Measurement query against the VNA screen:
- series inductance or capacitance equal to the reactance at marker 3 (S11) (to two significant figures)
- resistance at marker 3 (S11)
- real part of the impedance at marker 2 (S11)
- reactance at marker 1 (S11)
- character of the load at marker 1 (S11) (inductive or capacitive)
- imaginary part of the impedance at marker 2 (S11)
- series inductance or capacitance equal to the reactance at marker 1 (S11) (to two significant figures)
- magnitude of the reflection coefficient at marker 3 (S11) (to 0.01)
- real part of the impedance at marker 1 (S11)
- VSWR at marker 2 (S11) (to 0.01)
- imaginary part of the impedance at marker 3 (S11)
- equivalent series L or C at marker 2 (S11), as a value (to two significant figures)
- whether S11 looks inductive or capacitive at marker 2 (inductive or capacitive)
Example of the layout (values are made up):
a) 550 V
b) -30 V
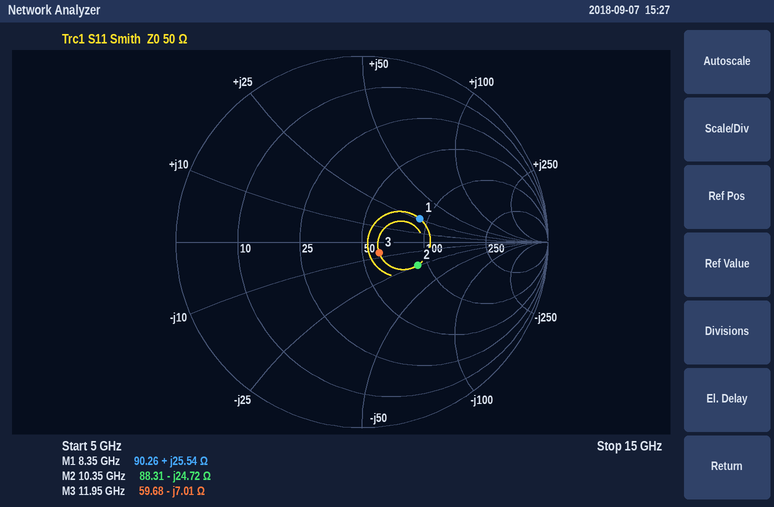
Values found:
a) 1.9 pF
b) 59.68 Ω
c) 88.31 Ω
d) +25.54 Ω
e) inductive
f) -24.72 Ω
g) 490 pH
h) 0.11
i) 90.26 Ω
j) 1.96
k) -7.01 Ω
l) 620 fF
m) capacitive
